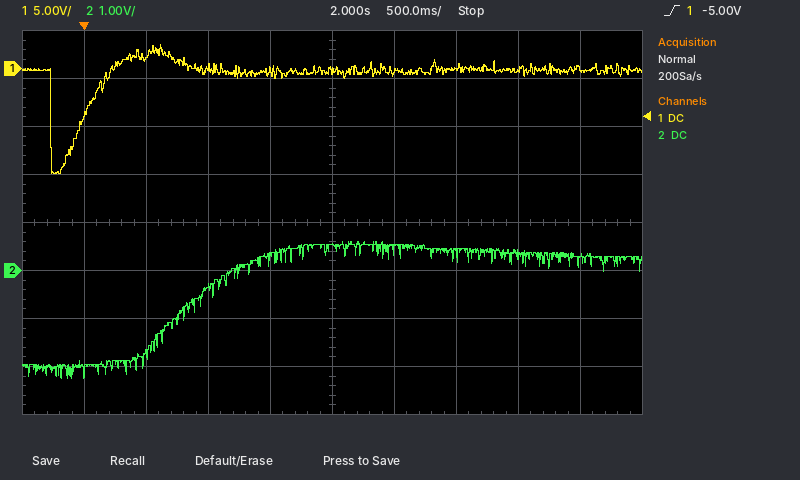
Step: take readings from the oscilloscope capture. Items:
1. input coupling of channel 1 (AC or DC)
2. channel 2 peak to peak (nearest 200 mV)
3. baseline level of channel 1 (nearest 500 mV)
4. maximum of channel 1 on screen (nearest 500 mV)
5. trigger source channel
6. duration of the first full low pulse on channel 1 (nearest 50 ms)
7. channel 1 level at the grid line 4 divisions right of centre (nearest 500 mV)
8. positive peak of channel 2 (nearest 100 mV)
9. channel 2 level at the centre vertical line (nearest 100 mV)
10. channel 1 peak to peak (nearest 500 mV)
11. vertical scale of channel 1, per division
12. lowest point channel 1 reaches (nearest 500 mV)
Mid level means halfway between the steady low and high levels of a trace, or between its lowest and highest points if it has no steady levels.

DC
2.8 V
0.0 V
2.5 V
channel 1
300 ms
0.0 V
600 mV
500 mV
13.5 V
5 V
-11.0 V
